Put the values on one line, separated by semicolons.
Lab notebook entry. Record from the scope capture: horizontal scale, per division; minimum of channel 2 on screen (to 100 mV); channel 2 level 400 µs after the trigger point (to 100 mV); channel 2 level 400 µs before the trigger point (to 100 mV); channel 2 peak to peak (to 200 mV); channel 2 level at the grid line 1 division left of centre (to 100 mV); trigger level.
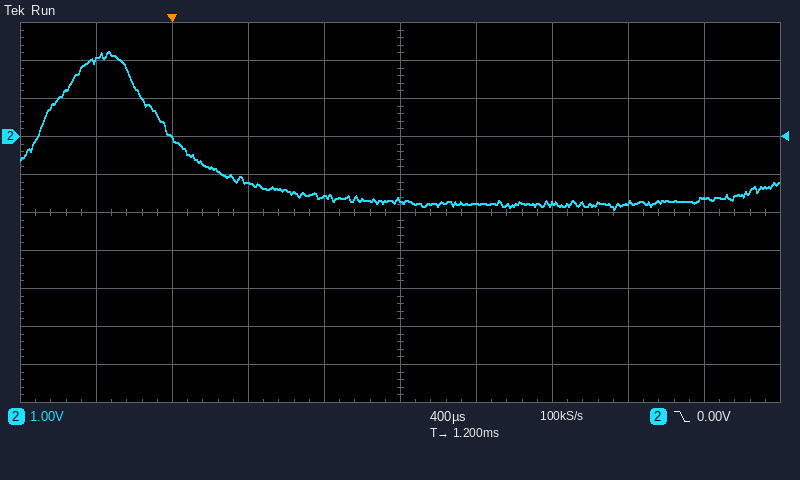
400 µs; -1.9 V; -1.2 V; 2.0 V; 4.2 V; -1.6 V; 0.00 V
